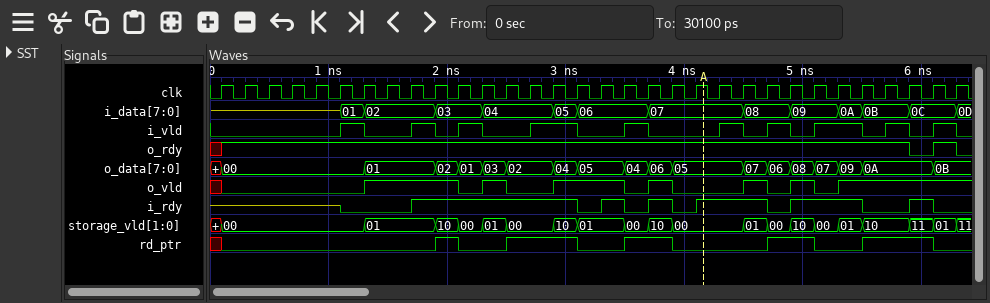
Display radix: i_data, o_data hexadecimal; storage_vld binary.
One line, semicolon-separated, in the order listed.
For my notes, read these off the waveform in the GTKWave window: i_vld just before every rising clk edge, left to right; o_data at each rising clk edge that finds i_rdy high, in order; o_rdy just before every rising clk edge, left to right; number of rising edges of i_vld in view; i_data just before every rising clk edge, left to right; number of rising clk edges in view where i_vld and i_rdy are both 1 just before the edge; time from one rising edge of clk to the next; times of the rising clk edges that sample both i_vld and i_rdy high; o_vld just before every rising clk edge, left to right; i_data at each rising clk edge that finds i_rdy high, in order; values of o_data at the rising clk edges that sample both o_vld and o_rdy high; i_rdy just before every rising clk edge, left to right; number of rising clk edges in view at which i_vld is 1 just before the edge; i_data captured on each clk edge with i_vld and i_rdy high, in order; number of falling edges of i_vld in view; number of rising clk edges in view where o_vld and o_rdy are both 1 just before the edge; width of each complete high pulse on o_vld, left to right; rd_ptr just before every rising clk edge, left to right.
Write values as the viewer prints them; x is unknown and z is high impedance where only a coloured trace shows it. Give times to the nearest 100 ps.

0 0 0 0 0 0 1 0 0 1 0 1 0 0 1 1 0 0 1 0 0 0 1 0 1 0 1 1 0 1 0 1; 01, 02, 01, 03, 02, 02, 04, 05, 06, 05, 05, 07, 08, 07, 09, 0A; x 1 1 1 1 1 1 1 1 1 1 1 1 1 1 1 1 1 1 1 1 1 1 1 1 1 1 1 1 1 0 1; 10; z, z, z, z, z, z, 01, 02, 02, 02, 03, 03, 04, 04, 04, 05, 06, 06, 06, 07, 07, 07, 07, 08, 08, 09, 09, 0A, 0B, 0B, 0C, 0C; 7; 200 ps; 1900 ps, 2300 ps, 2900 ps, 3100 ps, 4500 ps, 5300 ps, 5500 ps; x 0 0 0 0 0 0 1 1 1 1 0 1 0 0 1 1 1 0 1 0 0 0 1 0 1 0 1 1 1 1 1; 02, 03, 03, 04, 04, 04, 05, 06, 07, 07, 07, 08, 09, 09, 0A, 0C; 01, 01, 01, 02, 03, 04, 05, 05, 06, 07, 08, 09, 0A, 0A, 0B; z z z z z z 0 0 0 1 1 1 1 1 1 1 0 1 0 1 0 1 1 1 0 1 1 1 0 0 1 0; 12; 02, 03, 04, 05, 07, 09, 0A; 10; 15; 800 ps, 200 ps, 600 ps, 200 ps, 200 ps, 200 ps; x 0 0 0 0 0 0 0 0 0 1 0 0 1 1 1 0 0 1 1 0 0 0 0 1 1 0 0 1 1 1 0
